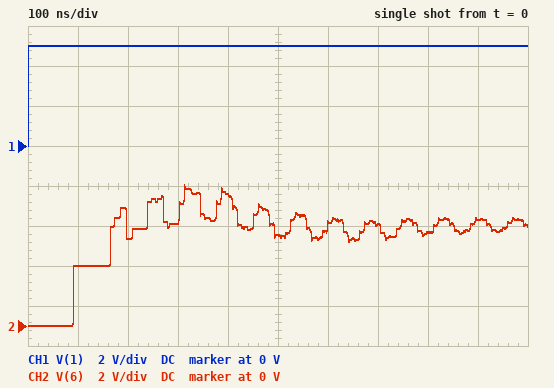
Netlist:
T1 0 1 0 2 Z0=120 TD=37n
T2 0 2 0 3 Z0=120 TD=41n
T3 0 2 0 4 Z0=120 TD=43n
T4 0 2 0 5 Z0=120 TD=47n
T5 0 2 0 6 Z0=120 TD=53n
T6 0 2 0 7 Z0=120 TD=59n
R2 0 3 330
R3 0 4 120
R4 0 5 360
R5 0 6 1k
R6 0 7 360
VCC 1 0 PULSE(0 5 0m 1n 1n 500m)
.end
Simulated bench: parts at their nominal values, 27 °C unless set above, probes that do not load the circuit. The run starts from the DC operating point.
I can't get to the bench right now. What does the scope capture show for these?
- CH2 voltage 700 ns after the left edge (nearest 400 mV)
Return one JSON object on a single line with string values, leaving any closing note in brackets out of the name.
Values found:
{"CH2 voltage 700 ns after the left edge": "5.2 V"}
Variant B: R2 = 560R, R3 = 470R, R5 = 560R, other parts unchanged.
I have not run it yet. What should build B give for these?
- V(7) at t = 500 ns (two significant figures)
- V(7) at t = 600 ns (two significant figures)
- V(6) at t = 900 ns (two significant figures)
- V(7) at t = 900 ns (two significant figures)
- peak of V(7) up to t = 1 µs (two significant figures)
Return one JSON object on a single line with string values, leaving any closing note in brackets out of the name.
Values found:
{"V(7) at t = 500 ns": "5.5 V", "V(7) at t = 600 ns": "4.2 V", "V(6) at t = 900 ns": "5.3 V", "V(7) at t = 900 ns": "5.1 V", "peak of V(7) up to t = 1 µs": "7.5 V"}
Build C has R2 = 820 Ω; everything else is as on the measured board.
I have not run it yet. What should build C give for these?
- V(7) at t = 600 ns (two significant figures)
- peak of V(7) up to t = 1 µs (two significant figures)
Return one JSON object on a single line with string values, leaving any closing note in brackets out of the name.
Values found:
{"V(7) at t = 600 ns": "4.5 V", "peak of V(7) up to t = 1 µs": "6.8 V"}
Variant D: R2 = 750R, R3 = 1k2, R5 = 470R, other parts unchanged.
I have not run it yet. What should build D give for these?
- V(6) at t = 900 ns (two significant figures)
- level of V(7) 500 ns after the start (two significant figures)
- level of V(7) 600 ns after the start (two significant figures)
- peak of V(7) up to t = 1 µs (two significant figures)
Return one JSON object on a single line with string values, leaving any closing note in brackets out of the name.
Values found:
{"V(6) at t = 900 ns": "5.4 V", "level of V(7) 500 ns after the start": "5.5 V", "level of V(7) 600 ns after the start": "4.0 V", "peak of V(7) up to t = 1 µs": "7.8 V"}
